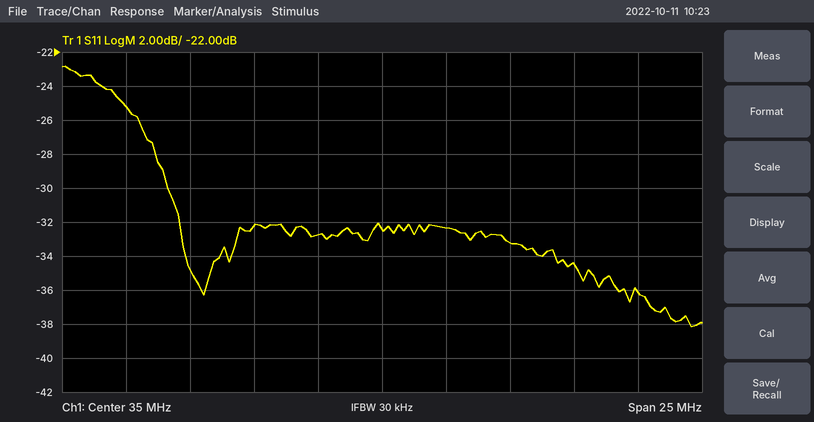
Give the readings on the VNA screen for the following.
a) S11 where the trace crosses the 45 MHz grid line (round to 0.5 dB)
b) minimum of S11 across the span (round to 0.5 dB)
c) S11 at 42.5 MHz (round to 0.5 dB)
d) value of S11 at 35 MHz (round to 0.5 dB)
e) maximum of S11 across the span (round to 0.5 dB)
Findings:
-36.0 dB
-38.0 dB
-34.5 dB
-32.5 dB
-23.0 dB
